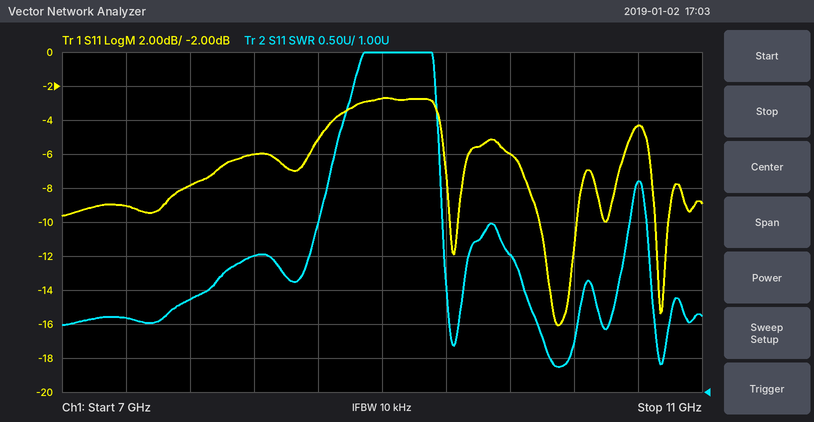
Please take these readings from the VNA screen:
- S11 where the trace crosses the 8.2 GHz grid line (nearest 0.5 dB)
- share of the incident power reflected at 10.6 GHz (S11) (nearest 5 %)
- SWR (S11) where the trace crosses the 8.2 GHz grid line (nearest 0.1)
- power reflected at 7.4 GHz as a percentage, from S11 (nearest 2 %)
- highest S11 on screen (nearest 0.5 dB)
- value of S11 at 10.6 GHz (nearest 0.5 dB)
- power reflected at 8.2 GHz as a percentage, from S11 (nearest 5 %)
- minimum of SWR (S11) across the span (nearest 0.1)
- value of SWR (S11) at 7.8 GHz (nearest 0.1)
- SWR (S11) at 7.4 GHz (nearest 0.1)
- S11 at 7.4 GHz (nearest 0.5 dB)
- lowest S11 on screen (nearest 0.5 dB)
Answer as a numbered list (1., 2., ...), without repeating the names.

1. -6.0 dB
2. 35 %
3. 3.0
4. 12 %
5. -2.5 dB
6. -4.5 dB
7. 25 %
8. 1.4
9. 2.4
10. 2.1
11. -9.0 dB
12. -16.0 dB
